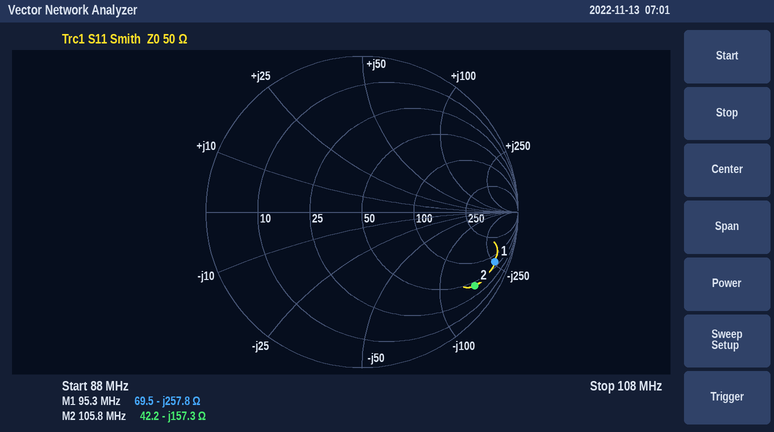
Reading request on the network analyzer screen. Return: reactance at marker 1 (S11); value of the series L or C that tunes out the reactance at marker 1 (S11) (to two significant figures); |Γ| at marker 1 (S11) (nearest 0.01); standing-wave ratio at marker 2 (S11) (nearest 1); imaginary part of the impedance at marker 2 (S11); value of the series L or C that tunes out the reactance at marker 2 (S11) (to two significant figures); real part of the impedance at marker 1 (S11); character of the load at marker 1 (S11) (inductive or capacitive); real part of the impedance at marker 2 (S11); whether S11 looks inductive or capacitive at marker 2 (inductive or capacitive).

-257.8 Ω
430 nH
0.91
14
-157.3 Ω
240 nH
69.5 Ω
capacitive
42.2 Ω
capacitive
